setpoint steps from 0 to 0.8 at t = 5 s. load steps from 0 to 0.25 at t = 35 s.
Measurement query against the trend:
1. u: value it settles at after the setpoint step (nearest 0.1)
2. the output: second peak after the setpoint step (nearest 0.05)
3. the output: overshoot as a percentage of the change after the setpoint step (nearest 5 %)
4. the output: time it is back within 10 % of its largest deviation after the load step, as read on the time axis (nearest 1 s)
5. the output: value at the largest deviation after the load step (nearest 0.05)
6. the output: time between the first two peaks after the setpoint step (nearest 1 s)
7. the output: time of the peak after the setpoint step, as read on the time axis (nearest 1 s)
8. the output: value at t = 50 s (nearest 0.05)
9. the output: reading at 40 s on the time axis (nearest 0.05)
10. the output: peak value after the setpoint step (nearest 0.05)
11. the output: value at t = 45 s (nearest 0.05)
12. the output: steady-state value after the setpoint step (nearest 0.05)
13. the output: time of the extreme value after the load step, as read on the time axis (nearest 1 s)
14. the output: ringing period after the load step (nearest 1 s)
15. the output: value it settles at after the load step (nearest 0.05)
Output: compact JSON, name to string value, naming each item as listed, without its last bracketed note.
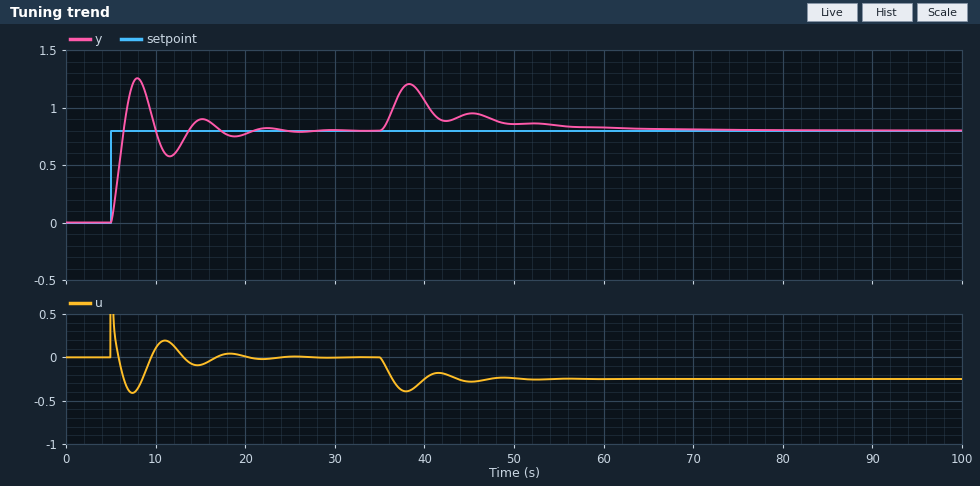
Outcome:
{"u: value it settles at after the setpoint step": "0.0", "the output: second peak after the setpoint step": "0.90", "the output: overshoot as a percentage of the change after the setpoint step": "55 %", "the output: time it is back within 10 % of its largest deviation after the load step, as read on the time axis": "55 s", "the output: value at the largest deviation after the load step": "1.20", "the output: time between the first two peaks after the setpoint step": "7 s", "the output: time of the peak after the setpoint step, as read on the time axis": "8 s", "the output: value at t = 50 s": "0.85", "the output: reading at 40 s on the time axis": "1.05", "the output: peak value after the setpoint step": "1.25", "the output: value at t = 45 s": "0.95", "the output: steady-state value after the setpoint step": "0.80", "the output: time of the extreme value after the load step, as read on the time axis": "38 s", "the output: ringing period after the load step": "7 s", "the output: value it settles at after the load step": "0.80"}
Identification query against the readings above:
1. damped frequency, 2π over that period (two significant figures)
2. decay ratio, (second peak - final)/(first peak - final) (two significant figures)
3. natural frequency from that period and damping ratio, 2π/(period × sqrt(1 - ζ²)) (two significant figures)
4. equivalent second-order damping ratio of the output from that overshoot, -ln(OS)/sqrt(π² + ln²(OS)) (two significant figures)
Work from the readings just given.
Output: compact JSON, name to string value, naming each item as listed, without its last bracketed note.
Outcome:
{"damped frequency, 2π over that period": "0.90 rad/s", "decay ratio, (second peak - final)/(first peak - final)": "0.22", "natural frequency from that period and damping ratio, 2π/(period × sqrt(1 - ζ²))": "0.91 rad/s", "equivalent second-order damping ratio of the output from that overshoot, -ln(OS)/sqrt(π² + ln²(OS))": "0.19"}
